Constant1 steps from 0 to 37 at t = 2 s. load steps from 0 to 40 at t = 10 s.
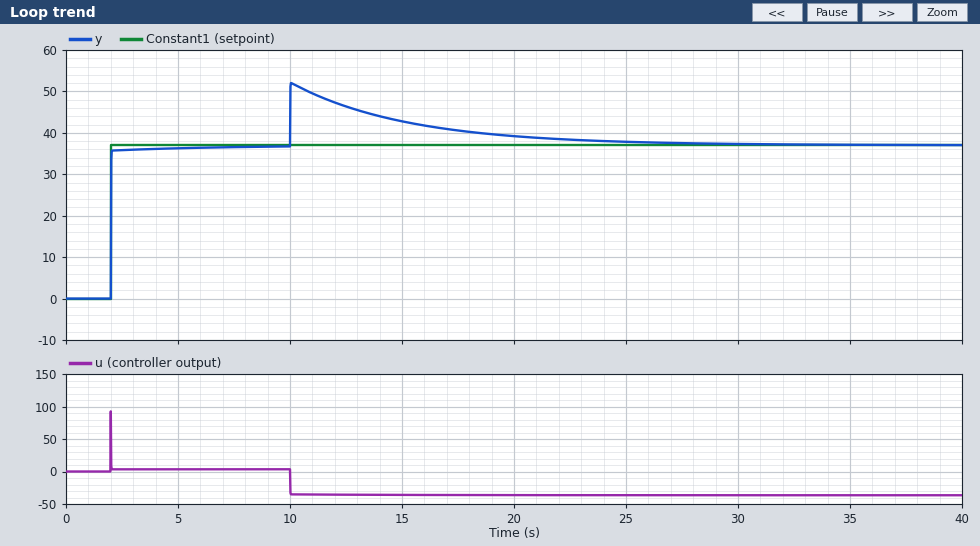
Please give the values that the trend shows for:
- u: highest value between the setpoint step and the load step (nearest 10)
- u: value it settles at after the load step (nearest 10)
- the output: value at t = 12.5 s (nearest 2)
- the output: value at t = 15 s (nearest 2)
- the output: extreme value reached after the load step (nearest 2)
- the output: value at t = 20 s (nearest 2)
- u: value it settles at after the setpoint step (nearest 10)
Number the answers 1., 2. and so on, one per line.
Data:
1. 90
2. -40
3. 46
4. 42
5. 52
6. 40
7. 0
